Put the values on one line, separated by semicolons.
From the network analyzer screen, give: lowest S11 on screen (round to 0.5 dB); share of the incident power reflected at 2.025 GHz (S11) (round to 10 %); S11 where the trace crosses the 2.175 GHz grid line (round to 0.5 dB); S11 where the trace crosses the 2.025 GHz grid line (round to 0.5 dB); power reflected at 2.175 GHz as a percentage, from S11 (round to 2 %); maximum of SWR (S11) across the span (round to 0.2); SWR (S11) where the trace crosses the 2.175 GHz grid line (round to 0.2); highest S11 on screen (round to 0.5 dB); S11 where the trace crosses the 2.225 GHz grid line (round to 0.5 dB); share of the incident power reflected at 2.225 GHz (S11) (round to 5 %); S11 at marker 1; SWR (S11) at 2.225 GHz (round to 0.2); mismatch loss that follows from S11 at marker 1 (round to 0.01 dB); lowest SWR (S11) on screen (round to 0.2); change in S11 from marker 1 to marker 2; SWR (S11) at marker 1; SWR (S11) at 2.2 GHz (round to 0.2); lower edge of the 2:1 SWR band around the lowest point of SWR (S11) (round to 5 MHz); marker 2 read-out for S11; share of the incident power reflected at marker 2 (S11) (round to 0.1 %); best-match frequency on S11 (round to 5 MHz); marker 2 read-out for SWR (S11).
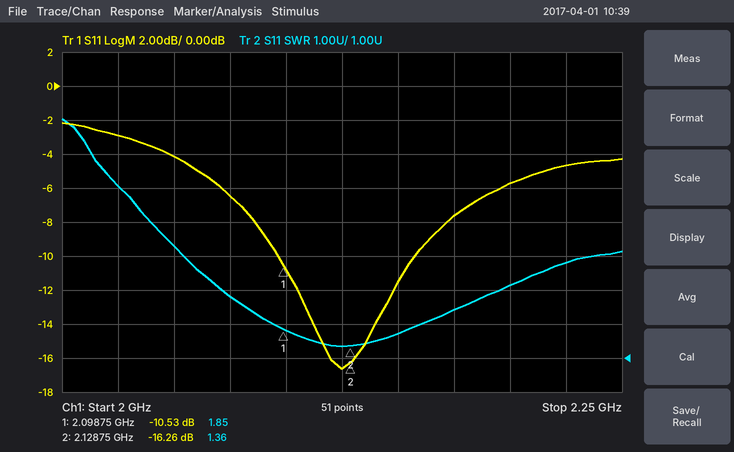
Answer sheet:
-16.5 dB; 50 %; -7.5 dB; -3.0 dB; 18 %; 8.0; 2.4; -2.0 dB; -4.5 dB; 35 %; -10.53 dB; 3.8; 0.40 dB; 1.4; -5.73 dB; 1.85; 3.2; 2.095 GHz; -16.26 dB; 2.4 %; 2.125 GHz; 1.36
